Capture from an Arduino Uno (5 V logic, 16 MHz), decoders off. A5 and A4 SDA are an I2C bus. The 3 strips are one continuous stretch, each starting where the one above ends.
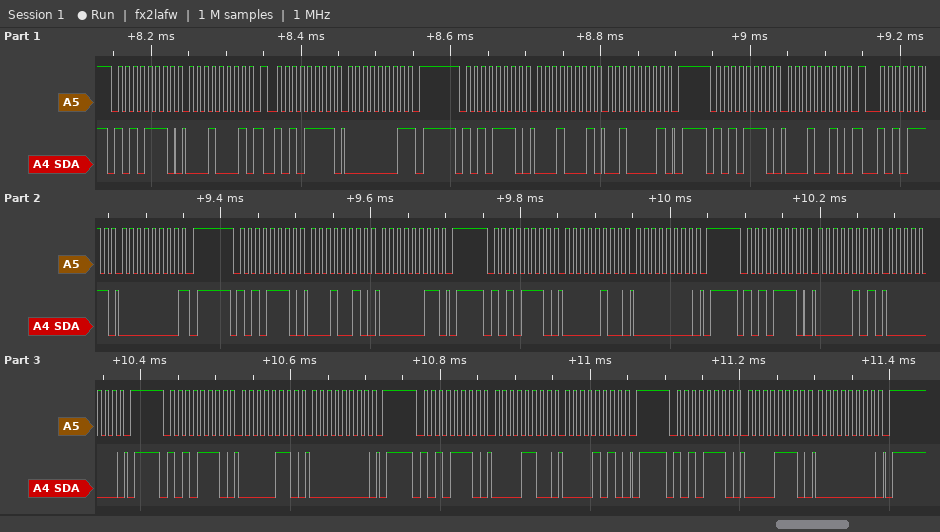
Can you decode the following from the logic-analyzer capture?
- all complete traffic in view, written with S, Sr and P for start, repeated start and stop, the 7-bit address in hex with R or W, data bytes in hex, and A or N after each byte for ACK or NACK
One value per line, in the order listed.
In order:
S 57W A 11 A Sr 57R A 01 N P S 57W A 11 A 21 A P S 57W A 12 A Sr 57R A 00 N P S 57W A 12 A 03 A P S 57W A 04 A 00 A P S 57W A 05 A 00 A P S 57W A 06 A 00 A P S 57W A 0C A 0A A P S 57W A 0E A 00 A P
